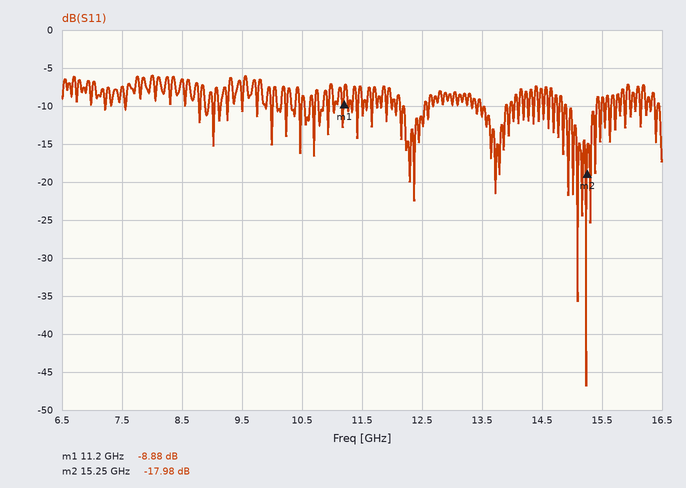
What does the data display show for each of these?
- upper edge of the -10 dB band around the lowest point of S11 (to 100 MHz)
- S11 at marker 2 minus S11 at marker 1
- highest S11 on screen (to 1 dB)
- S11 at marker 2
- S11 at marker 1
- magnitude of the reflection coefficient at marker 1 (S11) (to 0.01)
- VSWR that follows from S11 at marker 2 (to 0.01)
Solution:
15.4 GHz
-9.10 dB
-6 dB
-17.98 dB
-8.88 dB
0.36
1.29
